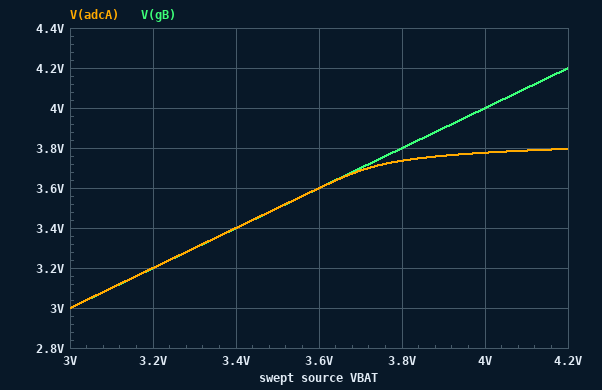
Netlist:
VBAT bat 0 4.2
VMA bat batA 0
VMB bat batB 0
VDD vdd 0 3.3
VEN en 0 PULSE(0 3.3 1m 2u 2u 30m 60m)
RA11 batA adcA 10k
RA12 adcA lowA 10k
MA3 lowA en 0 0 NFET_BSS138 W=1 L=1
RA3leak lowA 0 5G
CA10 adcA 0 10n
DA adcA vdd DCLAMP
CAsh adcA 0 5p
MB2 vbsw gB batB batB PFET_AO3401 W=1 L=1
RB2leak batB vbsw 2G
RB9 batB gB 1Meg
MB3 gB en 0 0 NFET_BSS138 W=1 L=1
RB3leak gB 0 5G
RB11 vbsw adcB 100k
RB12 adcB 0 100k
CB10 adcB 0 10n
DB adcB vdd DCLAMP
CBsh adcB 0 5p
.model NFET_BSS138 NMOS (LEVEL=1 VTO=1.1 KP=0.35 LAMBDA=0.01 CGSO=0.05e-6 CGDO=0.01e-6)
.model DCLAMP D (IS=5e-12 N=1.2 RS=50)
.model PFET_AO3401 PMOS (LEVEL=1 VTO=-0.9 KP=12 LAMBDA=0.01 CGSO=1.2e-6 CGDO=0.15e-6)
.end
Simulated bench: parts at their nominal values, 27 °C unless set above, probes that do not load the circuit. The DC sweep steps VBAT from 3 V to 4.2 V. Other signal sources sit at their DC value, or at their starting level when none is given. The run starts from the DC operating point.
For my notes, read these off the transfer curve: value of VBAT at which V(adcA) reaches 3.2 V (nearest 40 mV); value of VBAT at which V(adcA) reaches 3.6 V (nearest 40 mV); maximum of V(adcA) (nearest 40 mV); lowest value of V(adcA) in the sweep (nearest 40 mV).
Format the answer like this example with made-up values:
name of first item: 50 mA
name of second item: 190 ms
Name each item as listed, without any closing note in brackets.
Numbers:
value of VBAT at which V(adcA) reaches 3.2 V: 3.20 V
value of VBAT at which V(adcA) reaches 3.6 V: 3.60 V
maximum of V(adcA): 3.80 V
lowest value of V(adcA) in the sweep: 3.00 V
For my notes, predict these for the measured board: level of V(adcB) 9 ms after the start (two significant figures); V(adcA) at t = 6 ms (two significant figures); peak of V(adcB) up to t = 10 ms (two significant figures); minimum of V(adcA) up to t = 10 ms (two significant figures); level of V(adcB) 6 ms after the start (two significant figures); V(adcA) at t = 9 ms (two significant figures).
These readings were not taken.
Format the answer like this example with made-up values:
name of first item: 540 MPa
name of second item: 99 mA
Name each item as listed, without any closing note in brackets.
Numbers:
level of V(adcB) 9 ms after the start: 2.1 V
V(adcA) at t = 6 ms: 2.1 V
peak of V(adcB) up to t = 10 ms: 2.1 V
minimum of V(adcA) up to t = 10 ms: 2.1 V
level of V(adcB) 6 ms after the start: 2.1 V
V(adcA) at t = 9 ms: 2.1 V
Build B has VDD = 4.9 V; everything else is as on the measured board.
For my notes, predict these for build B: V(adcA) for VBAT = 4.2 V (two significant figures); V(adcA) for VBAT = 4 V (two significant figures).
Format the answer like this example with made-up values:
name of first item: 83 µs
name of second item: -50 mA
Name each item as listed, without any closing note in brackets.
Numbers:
V(adcA) for VBAT = 4.2 V: 4.2 V
V(adcA) for VBAT = 4 V: 4.0 V
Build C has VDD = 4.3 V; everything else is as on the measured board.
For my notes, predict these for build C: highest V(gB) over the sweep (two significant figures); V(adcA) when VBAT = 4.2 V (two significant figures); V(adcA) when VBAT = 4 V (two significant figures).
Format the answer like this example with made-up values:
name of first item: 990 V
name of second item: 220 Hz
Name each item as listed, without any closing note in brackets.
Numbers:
highest V(gB) over the sweep: 4.2 V
V(adcA) when VBAT = 4.2 V: 4.2 V
V(adcA) when VBAT = 4 V: 4.0 V
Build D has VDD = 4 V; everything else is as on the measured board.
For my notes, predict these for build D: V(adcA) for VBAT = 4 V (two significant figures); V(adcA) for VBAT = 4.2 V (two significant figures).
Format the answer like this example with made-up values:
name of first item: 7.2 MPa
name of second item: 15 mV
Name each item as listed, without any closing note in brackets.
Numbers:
V(adcA) for VBAT = 4 V: 4.0 V
V(adcA) for VBAT = 4.2 V: 4.2 V
